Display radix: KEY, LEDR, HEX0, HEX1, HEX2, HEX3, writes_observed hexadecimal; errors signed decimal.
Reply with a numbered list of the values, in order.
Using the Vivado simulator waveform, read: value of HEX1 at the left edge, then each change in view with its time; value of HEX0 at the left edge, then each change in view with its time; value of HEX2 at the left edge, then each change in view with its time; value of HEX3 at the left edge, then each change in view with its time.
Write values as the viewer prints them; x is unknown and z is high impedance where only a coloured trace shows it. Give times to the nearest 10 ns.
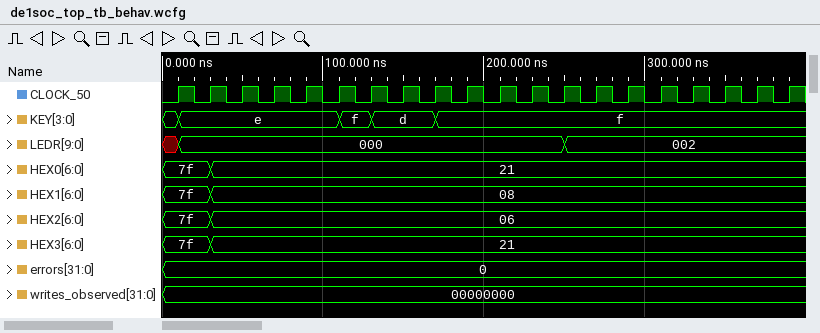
1. 7f, 08 at 30 ns
2. 7f, 21 at 30 ns
3. 7f, 06 at 30 ns
4. 7f, 21 at 30 ns
